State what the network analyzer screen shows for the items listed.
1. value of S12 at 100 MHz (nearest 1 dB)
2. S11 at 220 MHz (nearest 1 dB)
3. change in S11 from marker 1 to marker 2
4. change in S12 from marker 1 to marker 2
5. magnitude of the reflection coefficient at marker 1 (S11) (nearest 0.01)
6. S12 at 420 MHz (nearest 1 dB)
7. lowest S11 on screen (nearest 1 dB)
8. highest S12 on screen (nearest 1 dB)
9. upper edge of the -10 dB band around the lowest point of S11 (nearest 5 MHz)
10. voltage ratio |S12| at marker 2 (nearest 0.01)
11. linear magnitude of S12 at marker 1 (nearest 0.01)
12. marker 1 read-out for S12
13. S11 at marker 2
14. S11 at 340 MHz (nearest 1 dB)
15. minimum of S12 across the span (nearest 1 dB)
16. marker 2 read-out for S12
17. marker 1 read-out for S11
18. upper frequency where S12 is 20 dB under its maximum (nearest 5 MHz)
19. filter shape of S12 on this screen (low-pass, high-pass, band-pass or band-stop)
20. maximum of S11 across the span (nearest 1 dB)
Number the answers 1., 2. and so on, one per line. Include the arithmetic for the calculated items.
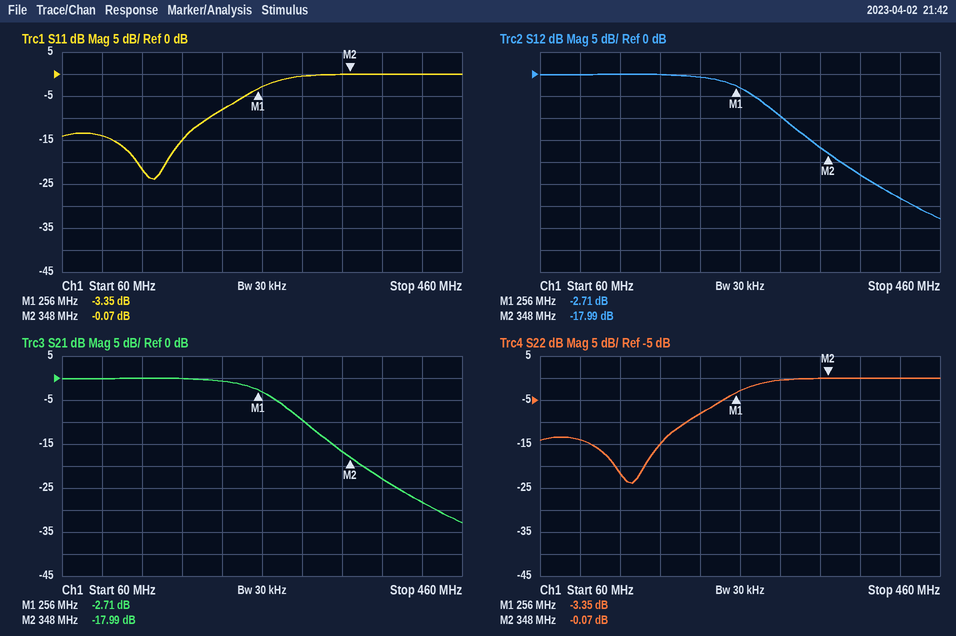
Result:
1. 0 dB
2. -8 dB
3. -0.07 − (-3.35) = 3.28 dB
4. -17.99 − (-2.71) = -15.28 dB
5. 10^(-3.35/20) ≈ 0.68
6. -28 dB
7. -24 dB
8. 0 dB
9. 205 MHz
10. 10^(-17.99/20) ≈ 0.13
11. 10^(-2.71/20) ≈ 0.73
12. -2.71 dB
13. -0.07 dB
14. 0 dB
15. -33 dB
16. -17.99 dB
17. -3.35 dB
18. 360 MHz
19. low-pass
20. 0 dB
